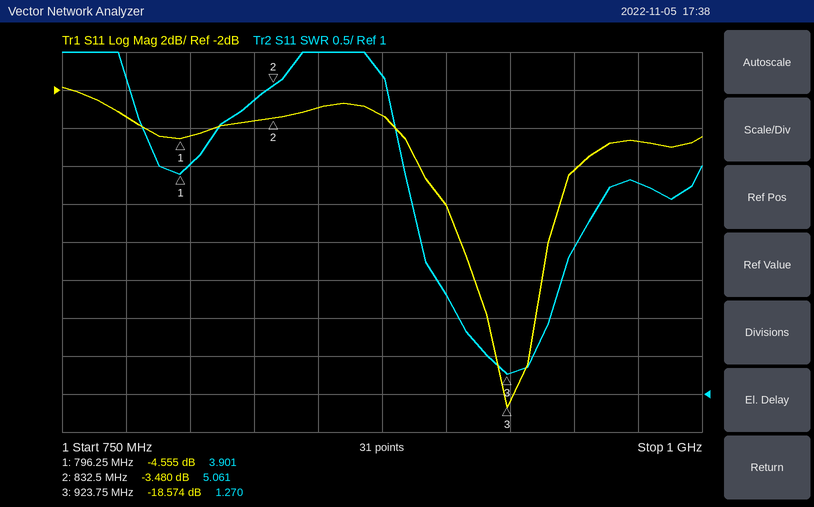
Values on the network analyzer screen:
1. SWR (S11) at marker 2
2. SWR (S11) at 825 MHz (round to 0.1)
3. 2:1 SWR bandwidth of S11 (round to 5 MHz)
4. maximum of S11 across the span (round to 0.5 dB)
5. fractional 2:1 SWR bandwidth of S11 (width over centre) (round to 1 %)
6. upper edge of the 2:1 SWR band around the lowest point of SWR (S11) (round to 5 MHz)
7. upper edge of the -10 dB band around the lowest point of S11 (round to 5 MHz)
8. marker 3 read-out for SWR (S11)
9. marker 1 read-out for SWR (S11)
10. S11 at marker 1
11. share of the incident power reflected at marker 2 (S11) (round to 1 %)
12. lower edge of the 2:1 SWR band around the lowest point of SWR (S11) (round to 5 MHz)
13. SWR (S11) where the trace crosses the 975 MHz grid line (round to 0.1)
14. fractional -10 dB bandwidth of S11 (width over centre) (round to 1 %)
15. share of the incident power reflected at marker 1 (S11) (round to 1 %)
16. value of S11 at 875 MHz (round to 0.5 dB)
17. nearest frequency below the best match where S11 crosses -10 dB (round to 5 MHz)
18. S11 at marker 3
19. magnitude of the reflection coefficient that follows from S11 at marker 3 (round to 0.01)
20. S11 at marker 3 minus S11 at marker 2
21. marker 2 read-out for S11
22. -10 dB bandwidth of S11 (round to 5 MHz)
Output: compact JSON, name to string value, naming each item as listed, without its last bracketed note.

{"SWR (S11) at marker 2": "5.061", "SWR (S11) at 825 MHz": "4.9", "2:1 SWR bandwidth of S11": "35 MHz", "maximum of S11 across the span": "-2.0 dB", "fractional 2:1 SWR bandwidth of S11 (width over centre)": "4 %", "upper edge of the 2:1 SWR band around the lowest point of SWR (S11)": "940 MHz", "upper edge of the -10 dB band around the lowest point of S11": "940 MHz", "marker 3 read-out for SWR": "1.270", "marker 1 read-out for SWR": "3.901", "S11 at marker 1": "-4.555 dB", "share of the incident power reflected at marker 2 (S11)": "45 %", "lower edge of the 2:1 SWR band around the lowest point of SWR (S11)": "905 MHz", "SWR (S11) where the trace crosses the 975 MHz grid line": "3.8", "fractional -10 dB bandwidth of S11 (width over centre)": "4 %", "share of the incident power reflected at marker 1 (S11)": "35 %", "value of S11 at 875 MHz": "-3.5 dB", "nearest frequency below the best match where S11 crosses -10 dB": "905 MHz", "S11 at marker 3": "-18.574 dB", "magnitude of the reflection coefficient that follows from S11 at marker 3": "0.12", "S11 at marker 3 minus S11 at marker 2": "-15.094 dB", "marker 2 read-out for S11": "-3.480 dB", "-10 dB bandwidth of S11": "35 MHz"}
